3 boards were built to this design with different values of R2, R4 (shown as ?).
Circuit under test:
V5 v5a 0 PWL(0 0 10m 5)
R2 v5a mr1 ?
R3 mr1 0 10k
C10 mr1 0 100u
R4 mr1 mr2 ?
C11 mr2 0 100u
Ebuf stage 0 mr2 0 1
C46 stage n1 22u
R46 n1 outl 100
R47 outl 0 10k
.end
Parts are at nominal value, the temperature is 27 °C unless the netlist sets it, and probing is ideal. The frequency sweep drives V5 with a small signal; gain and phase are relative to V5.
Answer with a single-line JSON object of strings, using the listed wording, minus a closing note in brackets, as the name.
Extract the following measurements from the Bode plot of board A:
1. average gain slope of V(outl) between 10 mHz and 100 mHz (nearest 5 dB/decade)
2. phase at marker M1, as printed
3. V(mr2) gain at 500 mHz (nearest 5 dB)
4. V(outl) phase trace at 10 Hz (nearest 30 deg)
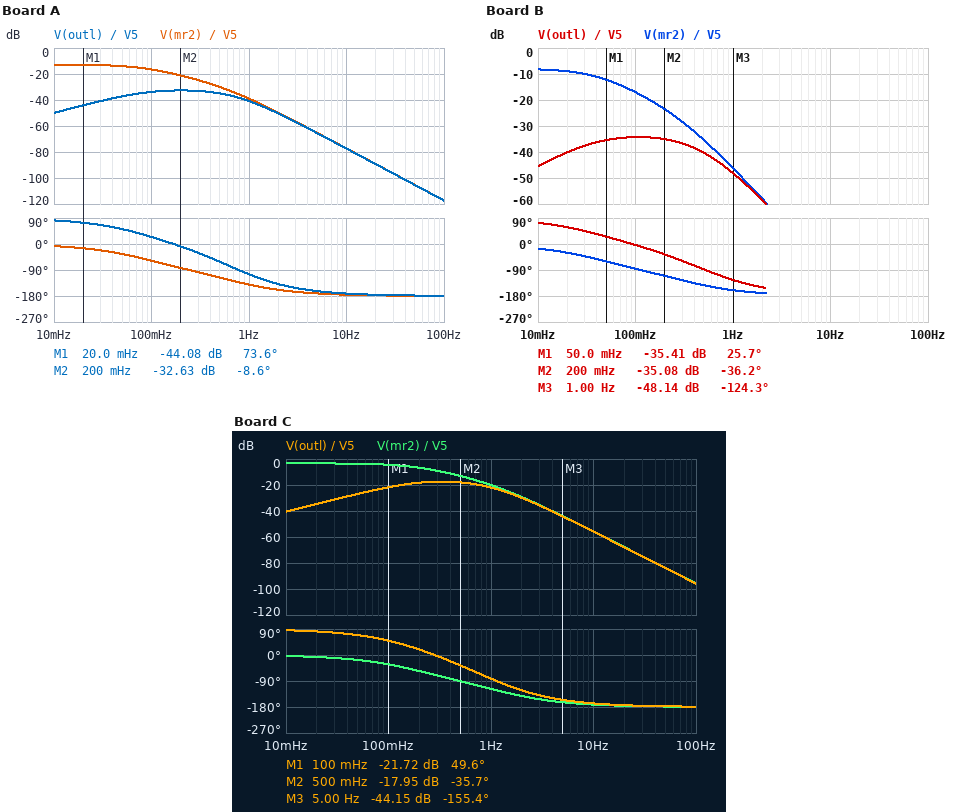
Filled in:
{"average gain slope of V(outl) between 10 mHz and 100 mHz": "15 dB/decade", "phase at marker M1, as printed": "73.6 deg", "V(mr2) gain at 500 mHz": "-30 dB", "V(outl) phase trace at 10 Hz": "-180 deg"}
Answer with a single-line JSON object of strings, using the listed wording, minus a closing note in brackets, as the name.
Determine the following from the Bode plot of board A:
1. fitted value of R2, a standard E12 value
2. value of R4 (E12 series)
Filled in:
{"fitted value of R2, a standard E12 value": "33 kΩ", "value of R4": "5.6 kΩ"}
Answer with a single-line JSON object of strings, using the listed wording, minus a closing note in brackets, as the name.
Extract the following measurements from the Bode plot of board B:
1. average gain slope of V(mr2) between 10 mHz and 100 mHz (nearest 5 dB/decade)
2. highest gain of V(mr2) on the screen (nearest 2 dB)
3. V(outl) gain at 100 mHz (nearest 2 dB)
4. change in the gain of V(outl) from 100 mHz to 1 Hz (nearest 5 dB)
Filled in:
{"average gain slope of V(mr2) between 10 mHz and 100 mHz": "-10 dB/decade", "highest gain of V(mr2) on the screen": "-8 dB", "V(outl) gain at 100 mHz": "-34 dB", "change in the gain of V(outl) from 100 mHz to 1 Hz": "-15 dB"}
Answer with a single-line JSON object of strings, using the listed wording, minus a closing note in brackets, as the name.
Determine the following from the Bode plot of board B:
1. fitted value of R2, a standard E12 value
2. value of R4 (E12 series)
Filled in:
{"fitted value of R2, a standard E12 value": "15 kΩ", "value of R4": "33 kΩ"}
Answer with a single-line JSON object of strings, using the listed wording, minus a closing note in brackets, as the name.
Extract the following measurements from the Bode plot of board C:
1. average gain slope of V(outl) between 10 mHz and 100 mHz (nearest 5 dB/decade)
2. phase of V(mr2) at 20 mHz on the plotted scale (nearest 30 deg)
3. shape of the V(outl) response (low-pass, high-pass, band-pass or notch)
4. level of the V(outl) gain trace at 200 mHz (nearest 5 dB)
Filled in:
{"average gain slope of V(outl) between 10 mHz and 100 mHz": "20 dB/decade", "phase of V(mr2) at 20 mHz on the plotted scale": "0 deg", "shape of the V(outl) response": "band-pass", "level of the V(outl) gain trace at 200 mHz": "-20 dB"}
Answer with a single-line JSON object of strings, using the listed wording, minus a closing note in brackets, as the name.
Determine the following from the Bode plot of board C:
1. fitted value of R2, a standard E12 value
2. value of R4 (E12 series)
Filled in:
{"fitted value of R2, a standard E12 value": "4.7 kΩ", "value of R4": "3.3 kΩ"}
